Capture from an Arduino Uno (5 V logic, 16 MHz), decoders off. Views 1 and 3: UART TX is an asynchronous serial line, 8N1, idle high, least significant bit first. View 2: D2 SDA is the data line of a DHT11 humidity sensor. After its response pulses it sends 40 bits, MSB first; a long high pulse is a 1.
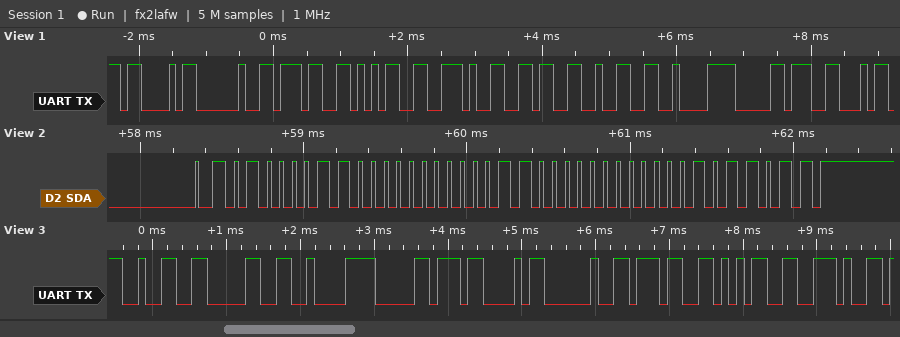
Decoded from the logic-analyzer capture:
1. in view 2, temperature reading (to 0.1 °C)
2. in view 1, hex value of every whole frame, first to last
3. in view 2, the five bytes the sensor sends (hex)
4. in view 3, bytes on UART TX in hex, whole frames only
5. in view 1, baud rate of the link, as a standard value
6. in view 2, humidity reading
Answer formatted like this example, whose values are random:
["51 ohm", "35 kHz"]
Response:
["24.0 °C", "43 20 37 35 2E 36 32 C2 B0 46", "43 00 18 00 5B", "32 30 C2 B0 43 20 37 35 2E", "9600 baud", "67 %"]
